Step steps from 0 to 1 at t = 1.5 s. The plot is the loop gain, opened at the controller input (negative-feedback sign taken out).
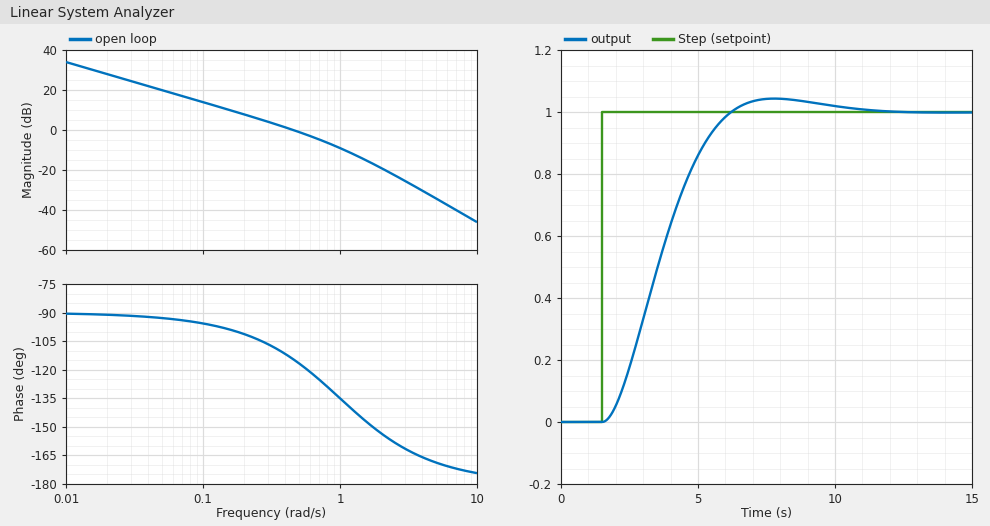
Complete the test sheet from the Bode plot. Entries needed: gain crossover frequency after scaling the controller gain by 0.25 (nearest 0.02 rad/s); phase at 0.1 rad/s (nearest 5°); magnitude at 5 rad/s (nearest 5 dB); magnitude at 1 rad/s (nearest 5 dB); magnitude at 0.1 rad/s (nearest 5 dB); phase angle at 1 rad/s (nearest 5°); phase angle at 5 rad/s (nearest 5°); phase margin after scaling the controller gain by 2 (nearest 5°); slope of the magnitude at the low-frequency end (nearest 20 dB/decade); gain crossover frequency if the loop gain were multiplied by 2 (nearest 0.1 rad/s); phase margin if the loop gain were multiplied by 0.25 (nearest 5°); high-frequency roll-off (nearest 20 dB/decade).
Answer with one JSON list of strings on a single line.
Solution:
["0.12 rad/s", "-95°", "-35 dB", "-10 dB", "15 dB", "-135°", "-170°", "50°", "-20 dB/decade", "0.8 rad/s", "85°", "-40 dB/decade"]
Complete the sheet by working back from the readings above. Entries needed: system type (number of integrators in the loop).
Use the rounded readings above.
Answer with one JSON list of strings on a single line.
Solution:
["1"]
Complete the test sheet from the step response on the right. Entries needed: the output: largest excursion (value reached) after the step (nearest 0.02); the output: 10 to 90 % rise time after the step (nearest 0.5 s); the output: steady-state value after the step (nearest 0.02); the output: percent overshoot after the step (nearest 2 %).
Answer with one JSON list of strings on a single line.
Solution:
["1.04", "3.0 s", "1.00", "4 %"]
